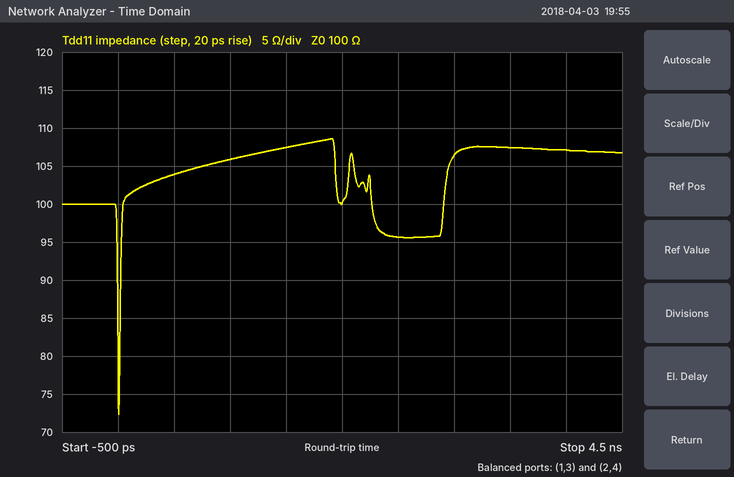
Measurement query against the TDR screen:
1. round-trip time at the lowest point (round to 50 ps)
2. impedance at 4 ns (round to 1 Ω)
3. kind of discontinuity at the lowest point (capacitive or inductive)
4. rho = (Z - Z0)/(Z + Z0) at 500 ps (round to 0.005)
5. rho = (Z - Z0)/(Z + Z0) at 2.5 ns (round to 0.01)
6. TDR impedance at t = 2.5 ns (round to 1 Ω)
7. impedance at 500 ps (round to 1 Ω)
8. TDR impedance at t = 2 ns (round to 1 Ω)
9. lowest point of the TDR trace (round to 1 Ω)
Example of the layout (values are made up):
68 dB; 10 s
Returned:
0 ps; 107 Ω; capacitive; +0.020; -0.02; 96 Ω; 104 Ω; 100 Ω; 72 Ω
